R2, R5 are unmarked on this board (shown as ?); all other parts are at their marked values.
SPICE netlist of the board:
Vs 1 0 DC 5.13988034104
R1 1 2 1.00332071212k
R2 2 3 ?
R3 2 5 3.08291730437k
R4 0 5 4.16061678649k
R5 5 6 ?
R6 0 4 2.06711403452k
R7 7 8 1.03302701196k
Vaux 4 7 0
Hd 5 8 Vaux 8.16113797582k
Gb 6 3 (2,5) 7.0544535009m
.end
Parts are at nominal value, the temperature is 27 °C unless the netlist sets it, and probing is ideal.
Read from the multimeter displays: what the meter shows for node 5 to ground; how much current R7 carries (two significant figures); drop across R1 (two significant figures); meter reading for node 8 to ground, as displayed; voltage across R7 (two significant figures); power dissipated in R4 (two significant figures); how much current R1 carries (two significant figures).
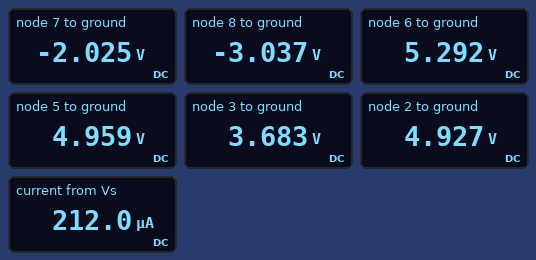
4.959 V
980 µA
210 mV
-3.037 V
1.0 V
5.9 mW
210 µA
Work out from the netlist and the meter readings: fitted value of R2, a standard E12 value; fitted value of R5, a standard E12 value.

5.6 kΩ
1.5 kΩ
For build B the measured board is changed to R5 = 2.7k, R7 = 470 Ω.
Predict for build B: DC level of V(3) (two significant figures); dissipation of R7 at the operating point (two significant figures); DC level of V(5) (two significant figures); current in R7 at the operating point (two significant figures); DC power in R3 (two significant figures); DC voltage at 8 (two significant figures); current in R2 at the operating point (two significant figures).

3.0 V
350 µW
4.9 V
870 µA
670 nW
-2.2 V
320 µA
